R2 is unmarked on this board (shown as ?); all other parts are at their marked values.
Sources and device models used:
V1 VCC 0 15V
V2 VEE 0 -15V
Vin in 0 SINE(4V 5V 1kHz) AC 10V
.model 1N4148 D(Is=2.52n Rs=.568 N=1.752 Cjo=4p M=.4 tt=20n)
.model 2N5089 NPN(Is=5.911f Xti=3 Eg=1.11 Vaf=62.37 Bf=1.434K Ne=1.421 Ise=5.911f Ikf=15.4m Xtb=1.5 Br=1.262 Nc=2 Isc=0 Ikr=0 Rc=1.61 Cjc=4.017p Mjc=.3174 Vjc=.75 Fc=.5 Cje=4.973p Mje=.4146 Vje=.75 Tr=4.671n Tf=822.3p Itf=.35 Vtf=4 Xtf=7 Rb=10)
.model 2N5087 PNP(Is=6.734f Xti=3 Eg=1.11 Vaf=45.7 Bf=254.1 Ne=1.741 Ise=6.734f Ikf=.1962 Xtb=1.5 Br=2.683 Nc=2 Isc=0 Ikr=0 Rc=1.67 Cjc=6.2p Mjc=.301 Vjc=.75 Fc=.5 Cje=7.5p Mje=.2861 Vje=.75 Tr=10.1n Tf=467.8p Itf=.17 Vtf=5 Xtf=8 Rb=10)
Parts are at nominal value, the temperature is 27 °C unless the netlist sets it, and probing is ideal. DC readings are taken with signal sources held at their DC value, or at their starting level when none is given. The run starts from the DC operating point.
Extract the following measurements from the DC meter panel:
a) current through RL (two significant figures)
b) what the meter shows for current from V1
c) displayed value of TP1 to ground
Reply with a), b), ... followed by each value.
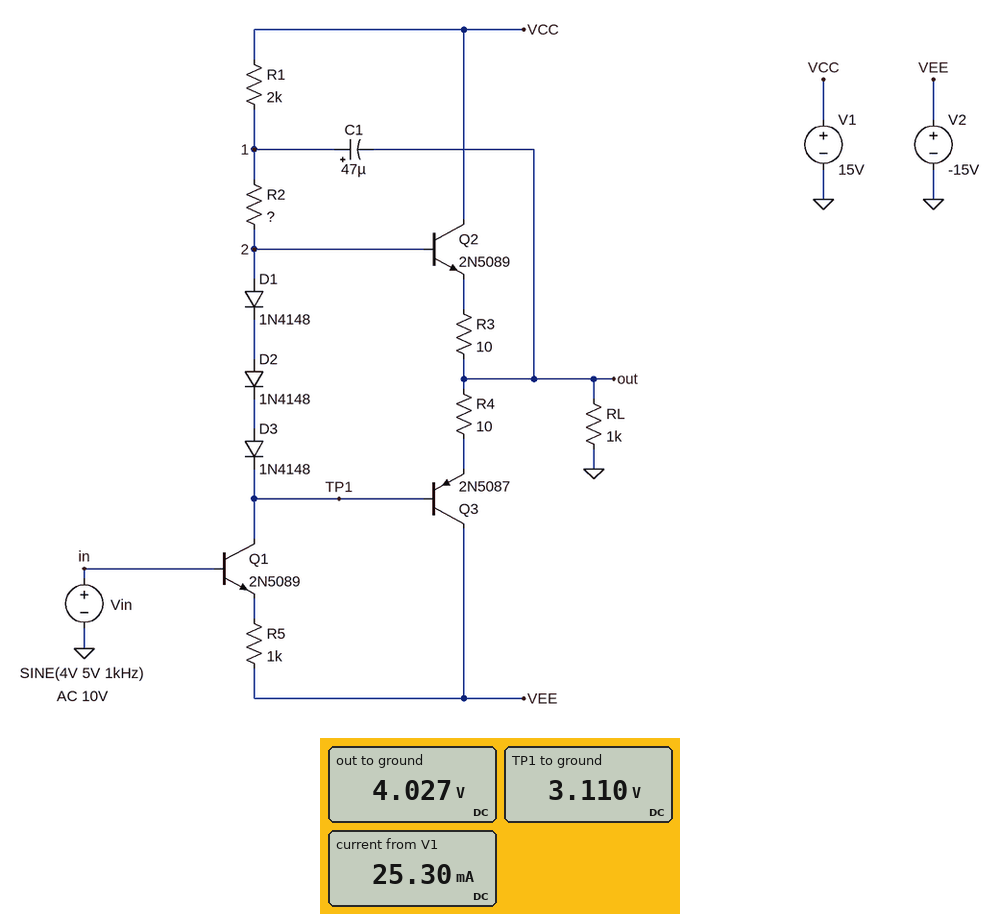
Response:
a) 4.0 mA
b) 25.30 mA
c) 3.110 V
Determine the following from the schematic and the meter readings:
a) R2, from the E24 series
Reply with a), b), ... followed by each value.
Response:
a) 1.3 kΩ
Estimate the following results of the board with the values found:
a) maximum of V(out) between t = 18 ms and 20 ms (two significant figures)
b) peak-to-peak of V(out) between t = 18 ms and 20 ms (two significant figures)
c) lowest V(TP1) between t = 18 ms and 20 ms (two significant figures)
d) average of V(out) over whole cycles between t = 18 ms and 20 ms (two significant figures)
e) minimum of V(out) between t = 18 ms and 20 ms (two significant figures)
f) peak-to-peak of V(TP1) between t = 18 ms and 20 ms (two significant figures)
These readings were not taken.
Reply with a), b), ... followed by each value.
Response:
a) 8.9 V
b) 9.8 V
c) -1.8 V
d) 4.0 V
e) -870 mV
f) 9.9 V
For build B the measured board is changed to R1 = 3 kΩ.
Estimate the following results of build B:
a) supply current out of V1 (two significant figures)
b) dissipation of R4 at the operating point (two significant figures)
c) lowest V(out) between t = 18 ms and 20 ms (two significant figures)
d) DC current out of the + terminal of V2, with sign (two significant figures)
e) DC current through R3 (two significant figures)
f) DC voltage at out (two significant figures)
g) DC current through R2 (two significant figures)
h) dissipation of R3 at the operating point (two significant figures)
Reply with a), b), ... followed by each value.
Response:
a) 23 mA
b) 2.8 mW
c) -900 mV
d) -35 mA
e) 21 mA
f) 4.0 V
g) 2.3 mA
h) 4.3 mW
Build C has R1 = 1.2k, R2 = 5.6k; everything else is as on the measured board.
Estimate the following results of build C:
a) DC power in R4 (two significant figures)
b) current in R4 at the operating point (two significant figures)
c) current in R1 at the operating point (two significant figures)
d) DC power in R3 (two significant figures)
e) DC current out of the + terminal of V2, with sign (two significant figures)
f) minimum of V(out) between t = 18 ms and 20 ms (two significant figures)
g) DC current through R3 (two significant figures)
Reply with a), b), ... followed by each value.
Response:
a) 2.0 mW
b) 14 mA
c) 1.5 mA
d) 3.3 mW
e) -32 mA
f) -930 mV
g) 18 mA
